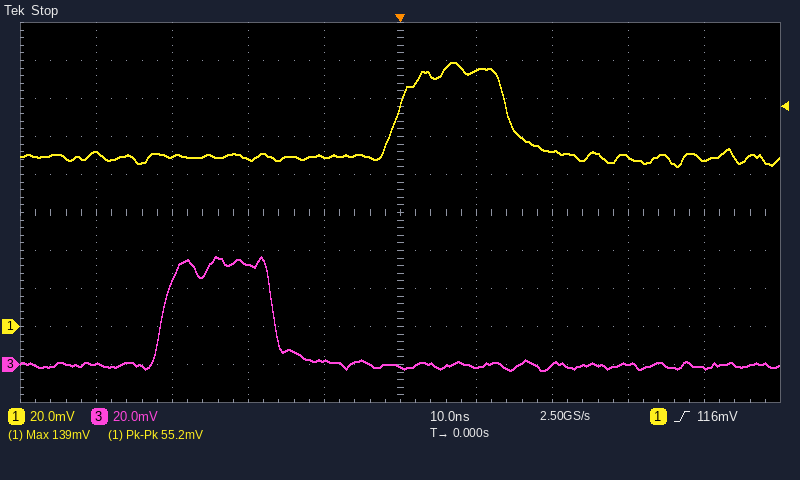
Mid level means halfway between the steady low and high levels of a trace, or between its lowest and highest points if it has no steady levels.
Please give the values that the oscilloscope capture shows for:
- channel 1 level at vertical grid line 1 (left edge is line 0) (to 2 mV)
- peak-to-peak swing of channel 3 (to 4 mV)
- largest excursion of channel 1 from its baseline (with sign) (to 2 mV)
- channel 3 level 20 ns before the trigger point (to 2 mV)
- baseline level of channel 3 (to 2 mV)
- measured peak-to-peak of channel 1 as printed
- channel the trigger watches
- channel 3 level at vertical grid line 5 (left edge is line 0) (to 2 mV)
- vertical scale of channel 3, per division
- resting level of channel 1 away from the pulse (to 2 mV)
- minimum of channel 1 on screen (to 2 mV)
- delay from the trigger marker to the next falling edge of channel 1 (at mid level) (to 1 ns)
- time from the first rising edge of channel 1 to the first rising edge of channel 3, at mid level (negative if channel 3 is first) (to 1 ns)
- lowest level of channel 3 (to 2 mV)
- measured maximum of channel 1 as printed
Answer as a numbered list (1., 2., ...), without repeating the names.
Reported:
1. 92 mV
2. 60 mV
3. +50 mV
4. 52 mV
5. 0 mV
6. 55.2 mV
7. channel 1
8. -2 mV
9. 20 mV
10. 90 mV
11. 84 mV
12. 14 ns
13. -31 ns
14. -4 mV
15. 139 mV
